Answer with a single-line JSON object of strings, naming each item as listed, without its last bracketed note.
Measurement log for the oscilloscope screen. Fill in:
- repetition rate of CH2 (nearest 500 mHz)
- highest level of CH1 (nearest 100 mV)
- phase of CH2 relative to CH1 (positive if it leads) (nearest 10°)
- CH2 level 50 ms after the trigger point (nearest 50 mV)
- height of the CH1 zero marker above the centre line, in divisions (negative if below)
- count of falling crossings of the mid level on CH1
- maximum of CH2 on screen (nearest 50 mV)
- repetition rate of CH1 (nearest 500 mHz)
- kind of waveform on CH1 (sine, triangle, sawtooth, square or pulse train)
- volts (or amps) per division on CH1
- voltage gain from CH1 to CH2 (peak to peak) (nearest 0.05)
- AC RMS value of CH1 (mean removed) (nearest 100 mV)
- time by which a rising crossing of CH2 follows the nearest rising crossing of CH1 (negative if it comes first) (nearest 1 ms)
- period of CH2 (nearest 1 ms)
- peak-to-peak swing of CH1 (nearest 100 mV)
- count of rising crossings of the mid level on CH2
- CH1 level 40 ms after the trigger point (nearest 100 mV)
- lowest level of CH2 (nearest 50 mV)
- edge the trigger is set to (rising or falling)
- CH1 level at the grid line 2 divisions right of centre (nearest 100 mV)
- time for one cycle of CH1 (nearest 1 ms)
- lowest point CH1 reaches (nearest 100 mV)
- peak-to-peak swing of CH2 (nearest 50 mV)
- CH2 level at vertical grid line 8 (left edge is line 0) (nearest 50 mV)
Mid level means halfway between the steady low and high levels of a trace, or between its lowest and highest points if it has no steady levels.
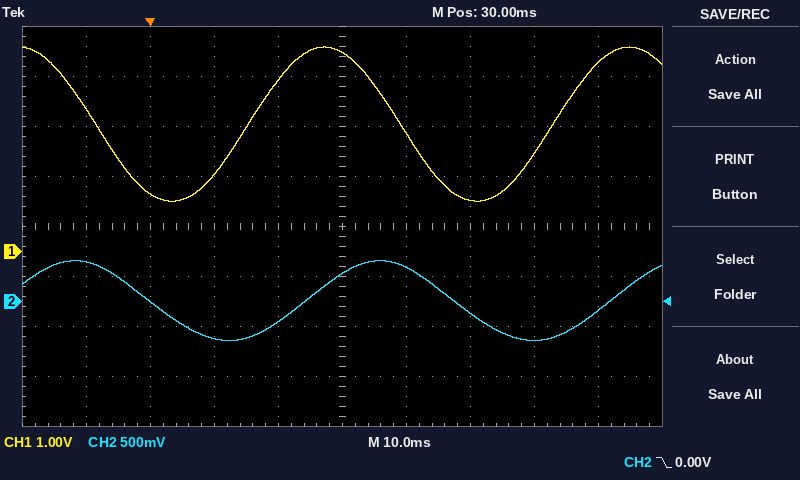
{"repetition rate of CH2": "21.0 Hz", "highest level of CH1": "4.1 V", "phase of CH2 relative to CH1 (positive if it leads)": "-70°", "CH2 level 50 ms after the trigger point": "-100 mV", "height of the CH1 zero marker above the centre line, in divisions": "-0.5 div", "count of falling crossings of the mid level on CH1": "2", "maximum of CH2 on screen": "400 mV", "repetition rate of CH1": "21.0 Hz", "kind of waveform on CH1": "sine", "volts (or amps) per division on CH1": "1 V", "voltage gain from CH1 to CH2 (peak to peak)": "0.25", "AC RMS value of CH1 (mean removed)": "1.1 V", "time by which a rising crossing of CH2 follows the nearest rising crossing of CH1 (negative if it comes first)": "+9 ms", "period of CH2": "48 ms", "peak-to-peak swing of CH1": "3.1 V", "count of rising crossings of the mid level on CH2": "2", "CH1 level 40 ms after the trigger point": "2.4 V", "lowest level of CH2": "-400 mV", "edge the trigger is set to": "falling", "CH1 level at the grid line 2 divisions right of centre": "1.0 V", "time for one cycle of CH1": "48 ms", "lowest point CH1 reaches": "1.0 V", "peak-to-peak swing of CH2": "800 mV", "CH2 level at vertical grid line 8 (left edge is line 0)": "-400 mV"}
